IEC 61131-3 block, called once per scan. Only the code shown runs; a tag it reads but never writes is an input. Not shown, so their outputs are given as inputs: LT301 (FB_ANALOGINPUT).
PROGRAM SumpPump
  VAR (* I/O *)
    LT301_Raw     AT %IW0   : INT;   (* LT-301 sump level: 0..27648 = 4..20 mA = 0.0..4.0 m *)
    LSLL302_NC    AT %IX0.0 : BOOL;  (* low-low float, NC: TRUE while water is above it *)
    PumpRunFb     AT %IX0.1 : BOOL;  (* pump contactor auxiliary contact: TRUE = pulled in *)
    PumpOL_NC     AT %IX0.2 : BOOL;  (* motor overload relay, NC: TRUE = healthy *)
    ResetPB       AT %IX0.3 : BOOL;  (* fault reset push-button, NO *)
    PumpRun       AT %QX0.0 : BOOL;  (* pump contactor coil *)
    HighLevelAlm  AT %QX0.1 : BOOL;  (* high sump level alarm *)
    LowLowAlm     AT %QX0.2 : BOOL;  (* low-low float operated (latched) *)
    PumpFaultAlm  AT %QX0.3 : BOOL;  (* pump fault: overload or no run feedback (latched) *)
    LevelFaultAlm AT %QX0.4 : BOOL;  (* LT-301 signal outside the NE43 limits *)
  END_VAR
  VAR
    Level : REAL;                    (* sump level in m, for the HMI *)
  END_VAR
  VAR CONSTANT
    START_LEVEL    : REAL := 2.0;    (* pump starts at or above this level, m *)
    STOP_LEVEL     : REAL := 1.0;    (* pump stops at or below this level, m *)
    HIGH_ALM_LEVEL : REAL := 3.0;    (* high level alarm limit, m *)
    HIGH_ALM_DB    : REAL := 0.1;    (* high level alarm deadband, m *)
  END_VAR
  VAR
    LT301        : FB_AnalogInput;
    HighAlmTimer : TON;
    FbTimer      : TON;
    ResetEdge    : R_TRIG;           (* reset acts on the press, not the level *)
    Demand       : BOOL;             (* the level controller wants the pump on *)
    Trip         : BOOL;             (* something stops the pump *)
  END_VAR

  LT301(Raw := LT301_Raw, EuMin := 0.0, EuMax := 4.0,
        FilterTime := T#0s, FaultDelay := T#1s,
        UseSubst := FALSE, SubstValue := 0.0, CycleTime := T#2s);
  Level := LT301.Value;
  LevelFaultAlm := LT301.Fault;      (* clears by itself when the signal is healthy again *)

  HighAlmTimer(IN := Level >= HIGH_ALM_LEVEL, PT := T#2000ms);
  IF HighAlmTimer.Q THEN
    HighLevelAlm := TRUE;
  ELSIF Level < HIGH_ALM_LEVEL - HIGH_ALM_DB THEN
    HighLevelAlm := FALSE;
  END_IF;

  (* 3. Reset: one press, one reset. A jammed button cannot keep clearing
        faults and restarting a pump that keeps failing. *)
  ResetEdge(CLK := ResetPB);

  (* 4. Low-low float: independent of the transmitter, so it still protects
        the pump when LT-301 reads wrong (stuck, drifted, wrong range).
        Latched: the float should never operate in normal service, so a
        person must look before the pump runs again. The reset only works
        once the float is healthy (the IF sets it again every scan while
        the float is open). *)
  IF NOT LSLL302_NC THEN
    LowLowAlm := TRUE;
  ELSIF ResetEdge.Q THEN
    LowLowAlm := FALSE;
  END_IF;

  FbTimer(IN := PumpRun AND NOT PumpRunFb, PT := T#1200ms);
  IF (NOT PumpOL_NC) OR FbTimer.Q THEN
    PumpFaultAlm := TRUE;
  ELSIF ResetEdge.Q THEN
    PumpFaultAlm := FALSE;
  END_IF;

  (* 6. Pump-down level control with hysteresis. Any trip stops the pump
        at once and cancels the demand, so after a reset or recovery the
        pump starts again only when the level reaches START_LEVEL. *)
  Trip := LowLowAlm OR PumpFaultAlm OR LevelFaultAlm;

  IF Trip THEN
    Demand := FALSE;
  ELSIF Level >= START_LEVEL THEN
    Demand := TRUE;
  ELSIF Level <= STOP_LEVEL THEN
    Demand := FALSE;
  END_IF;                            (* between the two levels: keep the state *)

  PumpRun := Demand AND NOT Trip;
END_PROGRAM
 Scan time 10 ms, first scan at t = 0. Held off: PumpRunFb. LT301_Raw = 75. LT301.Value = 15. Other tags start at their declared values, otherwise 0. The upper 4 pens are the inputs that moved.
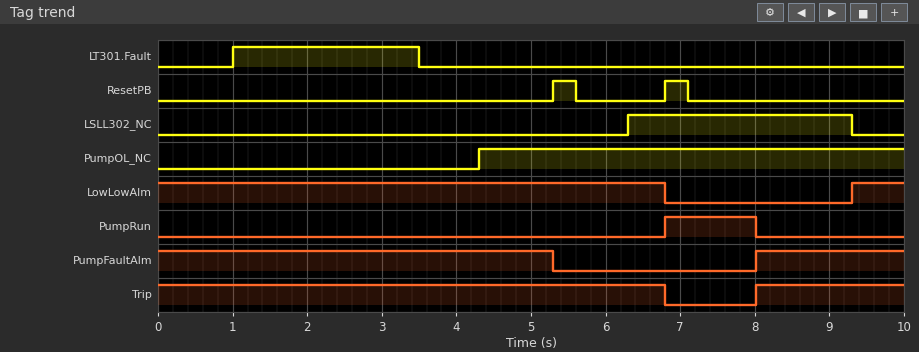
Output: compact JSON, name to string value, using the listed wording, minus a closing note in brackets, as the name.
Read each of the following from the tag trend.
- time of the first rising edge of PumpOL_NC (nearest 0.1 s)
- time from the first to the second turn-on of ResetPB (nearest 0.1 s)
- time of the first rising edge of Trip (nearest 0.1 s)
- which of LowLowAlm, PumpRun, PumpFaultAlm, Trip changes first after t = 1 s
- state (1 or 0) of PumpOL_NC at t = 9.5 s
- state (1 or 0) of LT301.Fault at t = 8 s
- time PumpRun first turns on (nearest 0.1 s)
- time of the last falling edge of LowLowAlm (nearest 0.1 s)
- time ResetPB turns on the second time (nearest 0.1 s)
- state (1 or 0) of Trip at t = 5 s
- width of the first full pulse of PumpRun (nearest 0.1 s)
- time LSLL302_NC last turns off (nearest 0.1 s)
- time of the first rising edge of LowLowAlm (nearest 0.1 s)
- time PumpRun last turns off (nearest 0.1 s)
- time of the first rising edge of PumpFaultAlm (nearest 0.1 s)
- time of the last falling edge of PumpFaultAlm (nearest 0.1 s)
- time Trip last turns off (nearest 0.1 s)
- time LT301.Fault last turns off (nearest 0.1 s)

{"time of the first rising edge of PumpOL_NC": "4.3 s", "time from the first to the second turn-on of ResetPB": "1.5 s", "time of the first rising edge of Trip": "8.0 s", "which of LowLowAlm, PumpRun, PumpFaultAlm, Trip changes first after t = 1 s": "PumpFaultAlm", "state (1 or 0) of PumpOL_NC at t = 9.5 s": "1", "state (1 or 0) of LT301.Fault at t = 8 s": "0", "time PumpRun first turns on": "6.8 s", "time of the last falling edge of LowLowAlm": "6.8 s", "time ResetPB turns on the second time": "6.8 s", "state (1 or 0) of Trip at t = 5 s": "1", "width of the first full pulse of PumpRun": "1.2 s", "time LSLL302_NC last turns off": "9.3 s", "time of the first rising edge of LowLowAlm": "9.3 s", "time PumpRun last turns off": "8.0 s", "time of the first rising edge of PumpFaultAlm": "8.0 s", "time of the last falling edge of PumpFaultAlm": "5.3 s", "time Trip last turns off": "6.8 s", "time LT301.Fault last turns off": "3.5 s"}
